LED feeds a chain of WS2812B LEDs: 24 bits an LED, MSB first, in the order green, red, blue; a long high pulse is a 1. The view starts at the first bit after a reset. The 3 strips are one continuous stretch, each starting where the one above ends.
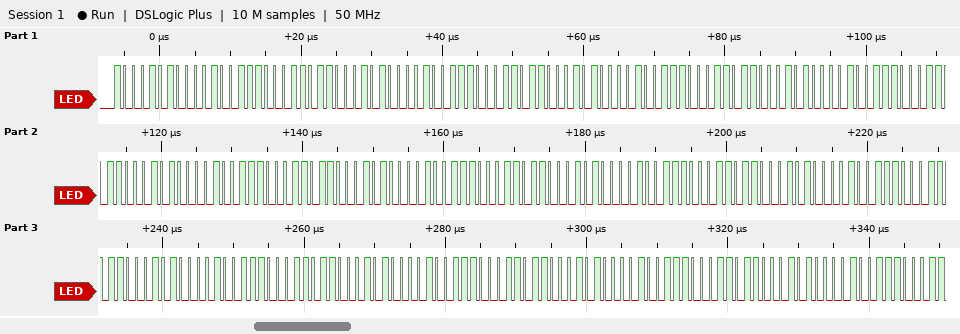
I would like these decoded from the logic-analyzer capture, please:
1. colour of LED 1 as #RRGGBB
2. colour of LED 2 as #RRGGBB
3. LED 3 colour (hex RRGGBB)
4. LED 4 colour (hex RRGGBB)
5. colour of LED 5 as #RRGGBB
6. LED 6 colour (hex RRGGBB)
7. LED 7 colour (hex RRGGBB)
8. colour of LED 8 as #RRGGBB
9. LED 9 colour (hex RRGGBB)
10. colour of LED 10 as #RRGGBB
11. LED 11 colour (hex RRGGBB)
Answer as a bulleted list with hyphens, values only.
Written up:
- #138A8D
- #138A8D
- #138A8D
- #138A8D
- #138A8D
- #138A8D
- #138A8D
- #138A8D
- #138A8D
- #138A8D
- #138A8D
